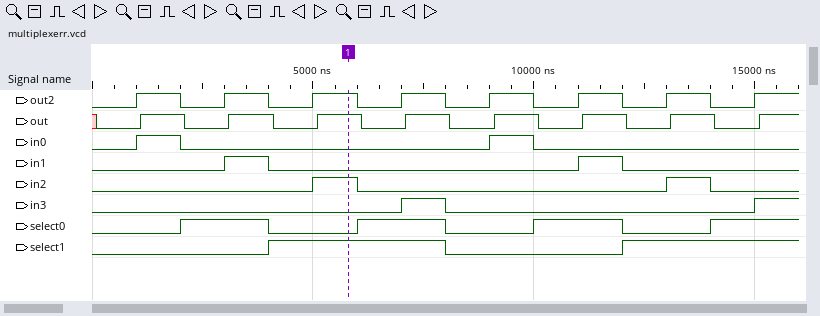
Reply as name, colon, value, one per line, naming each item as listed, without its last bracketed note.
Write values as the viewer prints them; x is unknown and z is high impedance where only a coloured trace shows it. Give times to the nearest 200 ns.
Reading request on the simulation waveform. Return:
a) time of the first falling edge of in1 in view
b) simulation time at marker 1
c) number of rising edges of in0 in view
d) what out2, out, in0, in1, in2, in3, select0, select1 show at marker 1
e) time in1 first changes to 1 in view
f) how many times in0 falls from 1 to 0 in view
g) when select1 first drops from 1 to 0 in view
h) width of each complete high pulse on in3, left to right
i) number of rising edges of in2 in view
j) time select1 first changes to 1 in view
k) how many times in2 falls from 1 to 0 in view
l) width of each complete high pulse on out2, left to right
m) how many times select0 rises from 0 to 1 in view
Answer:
time of the first falling edge of in1 in view: 4000 ns
simulation time at marker 1: 5800 ns
number of rising edges of in0 in view: 2
what out2, out, in0, in1, in2, in3, select0, select1 show at marker 1: out2=1, out=1, in0=0, in1=0, in2=1, in3=0, select0=0, select1=1
time in1 first changes to 1 in view: 3000 ns
how many times in0 falls from 1 to 0 in view: 2
when select1 first drops from 1 to 0 in view: 8000 ns
width of each complete high pulse on in3, left to right: 1000 ns
number of rising edges of in2 in view: 2
time select1 first changes to 1 in view: 4000 ns
how many times in2 falls from 1 to 0 in view: 2
width of each complete high pulse on out2, left to right: 1000 ns, 1000 ns, 1000 ns, 1000 ns, 1000 ns, 1000 ns, 1000 ns
how many times select0 rises from 0 to 1 in view: 4
